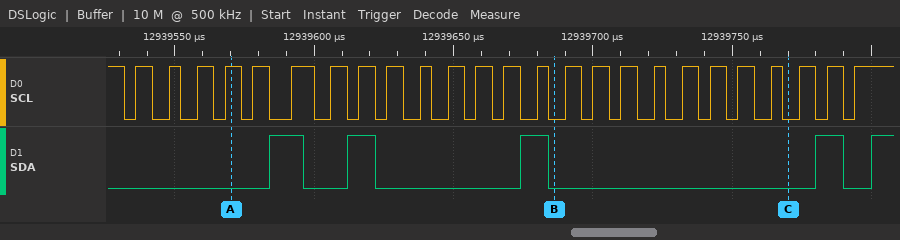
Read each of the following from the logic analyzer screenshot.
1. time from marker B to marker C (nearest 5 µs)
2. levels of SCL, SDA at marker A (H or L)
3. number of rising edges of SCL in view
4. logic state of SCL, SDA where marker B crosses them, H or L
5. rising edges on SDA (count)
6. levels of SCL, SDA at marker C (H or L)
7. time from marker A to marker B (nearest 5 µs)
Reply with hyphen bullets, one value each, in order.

- 85 µs
- SCL=H, SDA=L
- 25
- SCL=L, SDA=L
- 5
- SCL=L, SDA=L
- 115 µs
